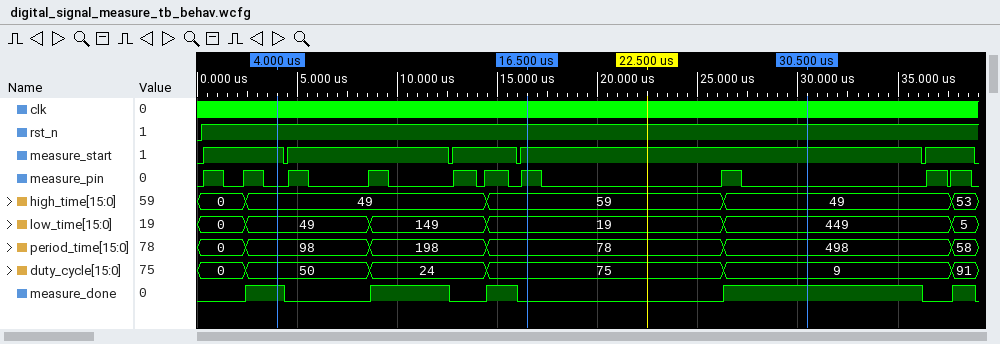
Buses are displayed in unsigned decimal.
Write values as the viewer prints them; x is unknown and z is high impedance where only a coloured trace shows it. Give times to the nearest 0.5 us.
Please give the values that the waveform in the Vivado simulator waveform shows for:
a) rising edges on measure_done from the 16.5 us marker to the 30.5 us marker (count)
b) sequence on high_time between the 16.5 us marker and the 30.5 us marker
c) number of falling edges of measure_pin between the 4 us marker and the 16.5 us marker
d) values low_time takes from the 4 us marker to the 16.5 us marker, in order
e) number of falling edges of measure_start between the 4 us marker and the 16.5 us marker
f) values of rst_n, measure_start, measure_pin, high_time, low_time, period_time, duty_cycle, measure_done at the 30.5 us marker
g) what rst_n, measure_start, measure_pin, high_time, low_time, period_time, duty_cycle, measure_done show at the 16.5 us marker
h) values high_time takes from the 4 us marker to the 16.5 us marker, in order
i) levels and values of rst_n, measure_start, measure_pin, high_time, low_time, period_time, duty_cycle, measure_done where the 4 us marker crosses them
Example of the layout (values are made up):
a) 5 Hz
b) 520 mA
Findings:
a) 1
b) 59, 49
c) 4
d) 49, 149, 19
e) 3
f) rst_n=1, measure_start=1, measure_pin=0, high_time=49, low_time=449, period_time=498, duty_cycle=9, measure_done=1
g) rst_n=1, measure_start=1, measure_pin=1, high_time=59, low_time=19, period_time=78, duty_cycle=75, measure_done=0
h) 49, 59
i) rst_n=1, measure_start=1, measure_pin=0, high_time=49, low_time=49, period_time=98, duty_cycle=50, measure_done=1
